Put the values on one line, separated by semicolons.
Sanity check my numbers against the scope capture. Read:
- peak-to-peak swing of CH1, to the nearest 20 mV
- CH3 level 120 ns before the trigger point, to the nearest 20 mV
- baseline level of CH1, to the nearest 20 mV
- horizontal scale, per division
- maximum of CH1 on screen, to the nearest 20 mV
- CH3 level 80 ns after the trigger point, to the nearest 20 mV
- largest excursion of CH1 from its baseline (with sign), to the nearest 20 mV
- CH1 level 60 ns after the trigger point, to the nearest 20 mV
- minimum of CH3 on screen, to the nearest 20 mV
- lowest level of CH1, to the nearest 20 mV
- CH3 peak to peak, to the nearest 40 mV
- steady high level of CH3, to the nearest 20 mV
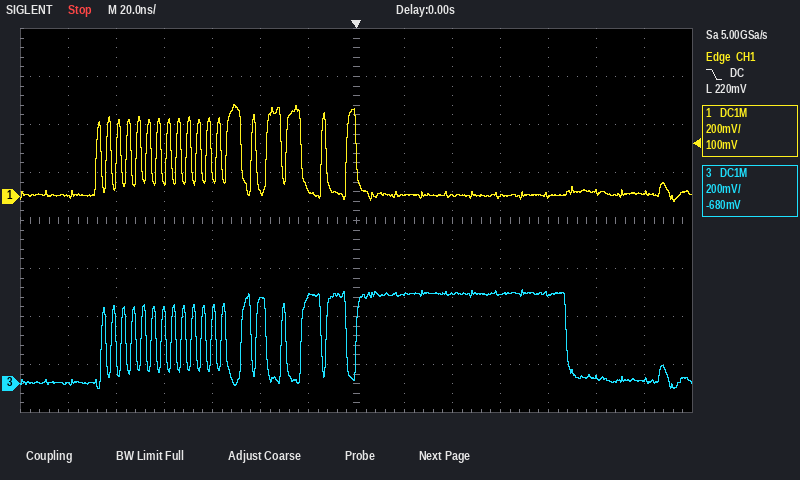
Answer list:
400 mV; 0 mV; 0 mV; 20 ns; 380 mV; 380 mV; +380 mV; 0 mV; -20 mV; -20 mV; 400 mV; 380 mV
